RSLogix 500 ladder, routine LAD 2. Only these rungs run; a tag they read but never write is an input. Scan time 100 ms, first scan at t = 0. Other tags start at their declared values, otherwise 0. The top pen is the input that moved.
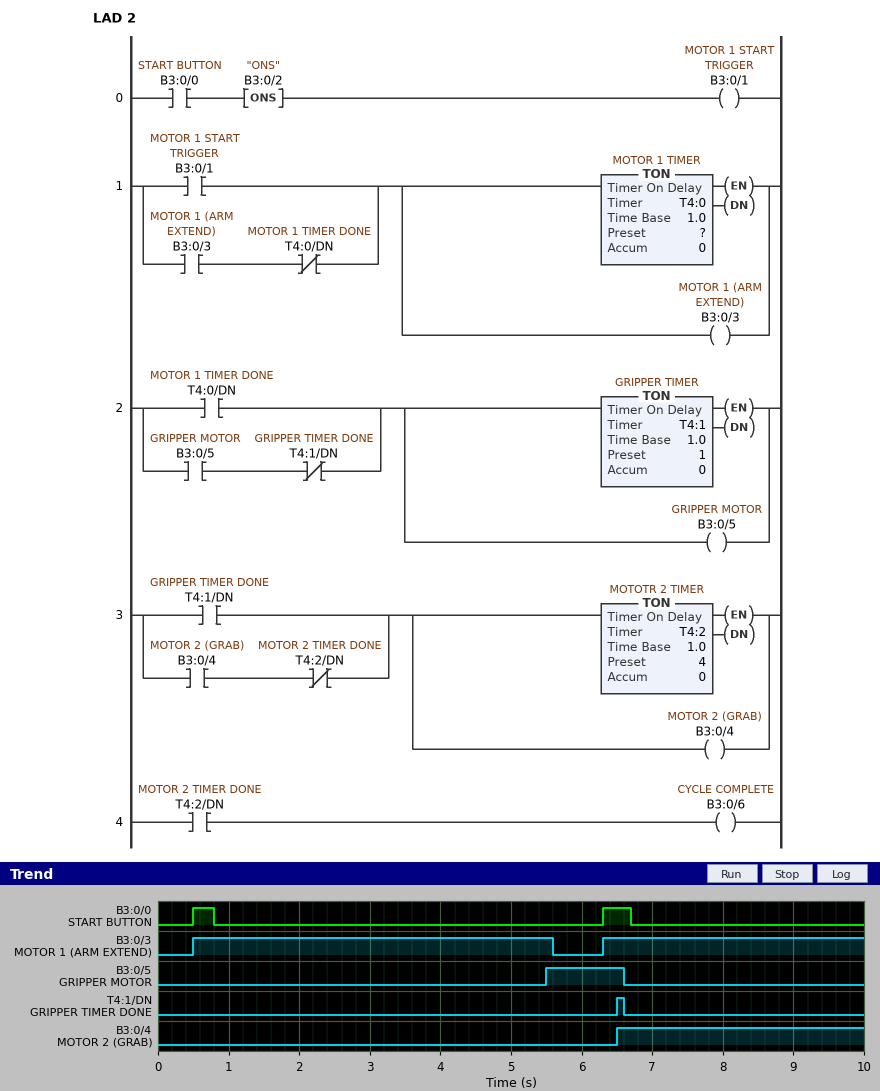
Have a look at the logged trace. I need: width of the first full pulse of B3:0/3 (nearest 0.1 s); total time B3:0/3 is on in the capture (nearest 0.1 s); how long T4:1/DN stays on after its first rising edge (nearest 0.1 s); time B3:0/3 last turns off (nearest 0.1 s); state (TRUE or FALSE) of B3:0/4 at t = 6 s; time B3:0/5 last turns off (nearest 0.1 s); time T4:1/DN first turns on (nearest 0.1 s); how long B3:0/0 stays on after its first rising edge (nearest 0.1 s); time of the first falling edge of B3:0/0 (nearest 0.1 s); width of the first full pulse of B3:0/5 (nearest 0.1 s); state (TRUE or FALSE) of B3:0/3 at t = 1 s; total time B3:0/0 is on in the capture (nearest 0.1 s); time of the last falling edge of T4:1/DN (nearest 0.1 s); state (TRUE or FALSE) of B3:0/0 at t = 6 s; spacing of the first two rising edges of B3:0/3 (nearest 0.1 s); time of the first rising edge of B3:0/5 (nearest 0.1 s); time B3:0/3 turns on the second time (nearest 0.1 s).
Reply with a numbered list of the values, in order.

1. 5.1 s
2. 8.8 s
3. 0.1 s
4. 5.6 s
5. FALSE
6. 6.6 s
7. 6.5 s
8. 0.3 s
9. 0.8 s
10. 1.1 s
11. TRUE
12. 0.7 s
13. 6.6 s
14. FALSE
15. 5.8 s
16. 5.5 s
17. 6.3 s
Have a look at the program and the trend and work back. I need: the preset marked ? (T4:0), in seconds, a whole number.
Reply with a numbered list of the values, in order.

1. 5 s
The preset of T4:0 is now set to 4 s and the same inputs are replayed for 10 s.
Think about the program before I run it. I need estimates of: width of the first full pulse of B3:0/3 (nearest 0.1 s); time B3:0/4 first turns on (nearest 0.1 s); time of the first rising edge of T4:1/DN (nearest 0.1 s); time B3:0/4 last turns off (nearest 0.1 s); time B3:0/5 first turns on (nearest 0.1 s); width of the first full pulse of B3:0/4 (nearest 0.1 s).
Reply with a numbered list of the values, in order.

1. 4.1 s
2. 5.5 s
3. 5.5 s
4. 9.6 s
5. 4.5 s
6. 4.1 s
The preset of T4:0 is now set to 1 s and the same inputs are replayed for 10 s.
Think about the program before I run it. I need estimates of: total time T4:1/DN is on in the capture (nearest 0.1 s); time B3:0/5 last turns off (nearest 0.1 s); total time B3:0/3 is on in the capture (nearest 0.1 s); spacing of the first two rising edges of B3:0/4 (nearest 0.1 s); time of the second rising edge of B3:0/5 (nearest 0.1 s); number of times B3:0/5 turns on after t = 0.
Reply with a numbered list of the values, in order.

1. 0.2 s
2. 8.4 s
3. 2.2 s
4. 5.8 s
5. 7.3 s
6. 2
